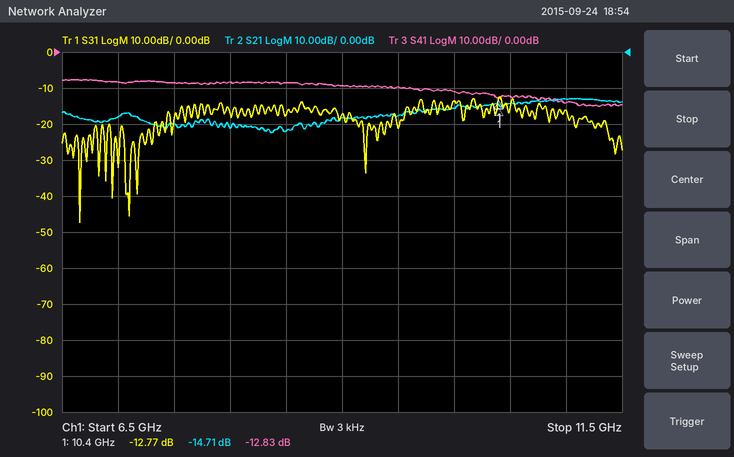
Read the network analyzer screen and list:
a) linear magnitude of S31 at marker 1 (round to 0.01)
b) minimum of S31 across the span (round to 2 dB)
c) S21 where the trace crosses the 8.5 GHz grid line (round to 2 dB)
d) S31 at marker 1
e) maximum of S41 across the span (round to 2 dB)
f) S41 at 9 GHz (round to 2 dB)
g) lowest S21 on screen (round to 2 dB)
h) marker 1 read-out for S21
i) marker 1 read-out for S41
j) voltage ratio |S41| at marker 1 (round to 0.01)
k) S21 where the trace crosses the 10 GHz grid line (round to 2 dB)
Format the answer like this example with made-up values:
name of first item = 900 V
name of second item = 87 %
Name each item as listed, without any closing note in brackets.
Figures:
linear magnitude of S31 at marker 1 = 0.23
minimum of S31 across the span = -48 dB
S21 where the trace crosses the 8.5 GHz grid line = -22 dB
S31 at marker 1 = -12.77 dB
maximum of S41 across the span = -8 dB
S41 at 9 GHz = -10 dB
lowest S21 on screen = -22 dB
marker 1 read-out for S21 = -14.71 dB
marker 1 read-out for S41 = -12.83 dB
voltage ratio |S41| at marker 1 = 0.23
S21 where the trace crosses the 10 GHz grid line = -16 dB
